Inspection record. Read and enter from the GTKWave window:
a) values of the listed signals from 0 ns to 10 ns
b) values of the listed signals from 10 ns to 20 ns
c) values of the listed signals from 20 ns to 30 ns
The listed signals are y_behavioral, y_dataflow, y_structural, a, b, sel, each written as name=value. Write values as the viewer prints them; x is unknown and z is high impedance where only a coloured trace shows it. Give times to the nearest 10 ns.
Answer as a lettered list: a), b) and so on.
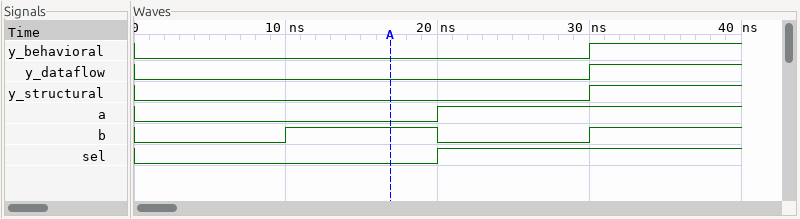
a) y_behavioral=0, y_dataflow=0, y_structural=0, a=0, b=0, sel=0
b) y_behavioral=0, y_dataflow=0, y_structural=0, a=0, b=1, sel=0
c) y_behavioral=0, y_dataflow=0, y_structural=0, a=1, b=0, sel=1
